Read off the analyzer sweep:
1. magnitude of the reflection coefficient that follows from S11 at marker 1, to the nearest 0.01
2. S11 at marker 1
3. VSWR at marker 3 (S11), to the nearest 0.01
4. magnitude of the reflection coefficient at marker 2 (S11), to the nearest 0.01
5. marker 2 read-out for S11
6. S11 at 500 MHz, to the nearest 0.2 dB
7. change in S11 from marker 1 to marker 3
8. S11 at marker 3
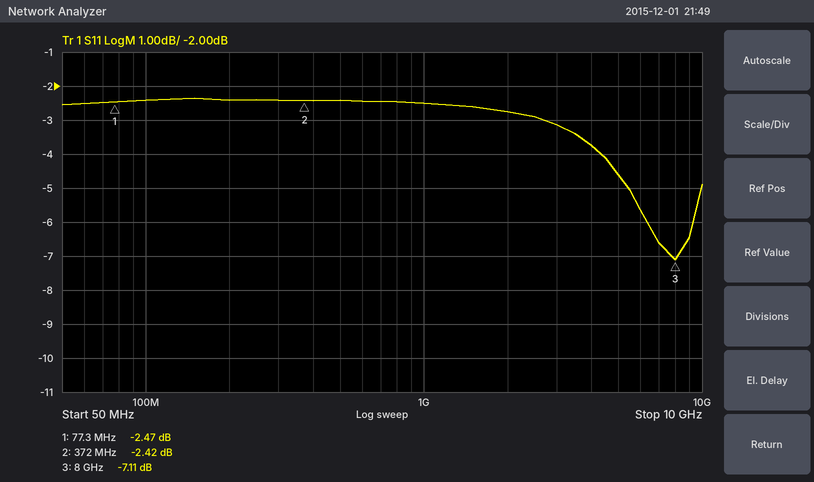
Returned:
0.75
-2.47 dB
2.58
0.76
-2.42 dB
-2.4 dB
-4.64 dB
-7.11 dB
